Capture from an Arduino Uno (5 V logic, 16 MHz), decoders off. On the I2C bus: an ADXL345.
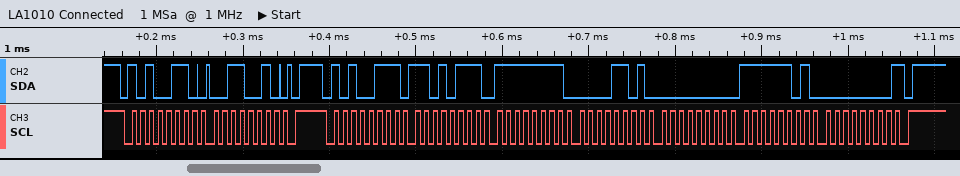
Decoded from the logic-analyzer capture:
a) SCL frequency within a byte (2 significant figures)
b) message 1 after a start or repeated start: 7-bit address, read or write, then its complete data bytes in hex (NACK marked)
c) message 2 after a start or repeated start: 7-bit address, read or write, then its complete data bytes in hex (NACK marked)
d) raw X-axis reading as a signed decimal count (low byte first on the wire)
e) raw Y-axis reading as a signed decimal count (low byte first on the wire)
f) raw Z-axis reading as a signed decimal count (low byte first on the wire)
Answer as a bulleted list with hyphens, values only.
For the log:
- 100 kHz
- 0x53 write: 32
- 0x53 read: D7 FF 0D 00 FD 00 NACK
- -41
- 13
- 253
